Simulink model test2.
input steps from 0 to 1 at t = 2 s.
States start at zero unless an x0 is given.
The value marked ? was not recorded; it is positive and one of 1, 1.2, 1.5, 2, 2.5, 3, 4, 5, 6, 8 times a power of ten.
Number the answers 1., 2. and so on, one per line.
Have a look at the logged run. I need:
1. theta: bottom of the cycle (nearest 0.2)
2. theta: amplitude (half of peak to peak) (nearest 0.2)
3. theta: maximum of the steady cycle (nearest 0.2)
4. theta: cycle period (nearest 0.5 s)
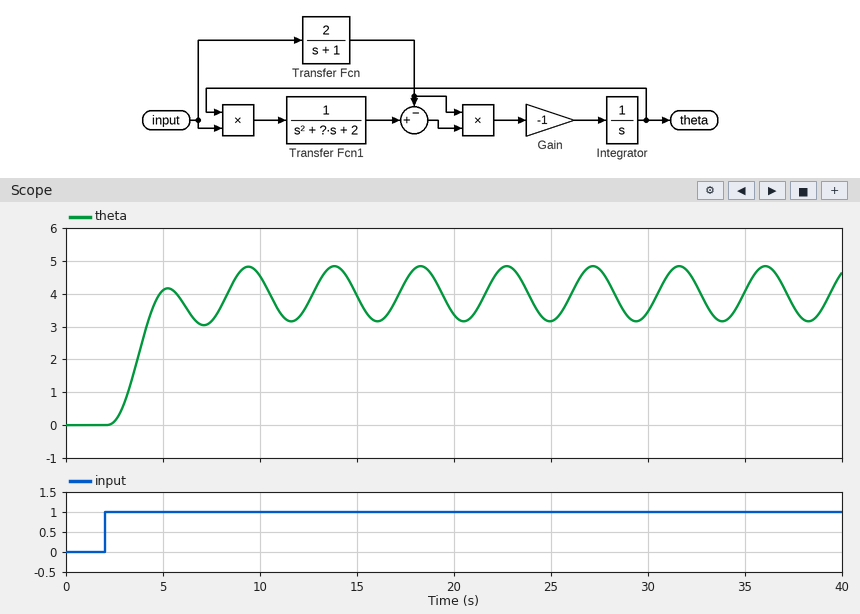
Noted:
1. 3.2
2. 0.8
3. 4.8
4. 4.5 s
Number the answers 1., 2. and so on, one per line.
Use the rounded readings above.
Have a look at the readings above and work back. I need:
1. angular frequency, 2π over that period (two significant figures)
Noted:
1. 1.4 rad/s
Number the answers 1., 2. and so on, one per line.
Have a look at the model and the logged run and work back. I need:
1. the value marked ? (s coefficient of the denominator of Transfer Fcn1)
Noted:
1. 1
